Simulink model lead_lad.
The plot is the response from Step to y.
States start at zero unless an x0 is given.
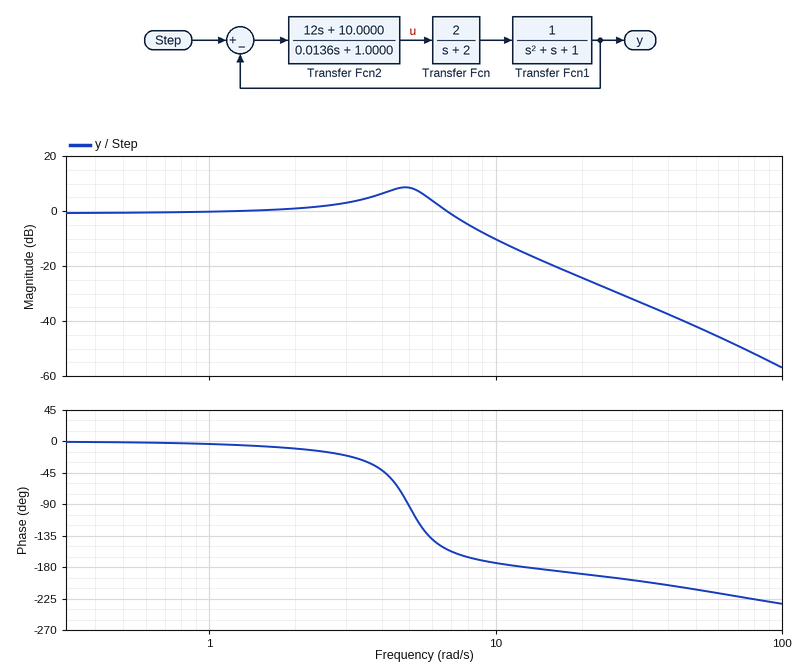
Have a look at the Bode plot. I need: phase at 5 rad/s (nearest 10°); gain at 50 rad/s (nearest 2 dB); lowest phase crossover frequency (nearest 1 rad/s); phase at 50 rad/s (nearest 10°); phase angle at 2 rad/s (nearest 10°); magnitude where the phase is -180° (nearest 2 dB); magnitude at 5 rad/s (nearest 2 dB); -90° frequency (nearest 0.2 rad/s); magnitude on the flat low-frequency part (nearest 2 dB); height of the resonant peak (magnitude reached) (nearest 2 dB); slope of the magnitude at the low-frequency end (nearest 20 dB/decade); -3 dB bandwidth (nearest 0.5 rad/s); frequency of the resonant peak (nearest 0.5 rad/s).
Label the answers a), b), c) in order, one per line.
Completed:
a) -90°
b) -42 dB
c) 13 rad/s
d) -210°
e) -10°
f) -16 dB
g) 8 dB
h) 5.0 rad/s
i) 0 dB
j) 8 dB
k) 0 dB/decade
l) 7.5 rad/s
m) 5.0 rad/s
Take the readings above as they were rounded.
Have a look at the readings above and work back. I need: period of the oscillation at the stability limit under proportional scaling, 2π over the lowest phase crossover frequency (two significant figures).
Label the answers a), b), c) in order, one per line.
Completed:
a) 0.48 s
